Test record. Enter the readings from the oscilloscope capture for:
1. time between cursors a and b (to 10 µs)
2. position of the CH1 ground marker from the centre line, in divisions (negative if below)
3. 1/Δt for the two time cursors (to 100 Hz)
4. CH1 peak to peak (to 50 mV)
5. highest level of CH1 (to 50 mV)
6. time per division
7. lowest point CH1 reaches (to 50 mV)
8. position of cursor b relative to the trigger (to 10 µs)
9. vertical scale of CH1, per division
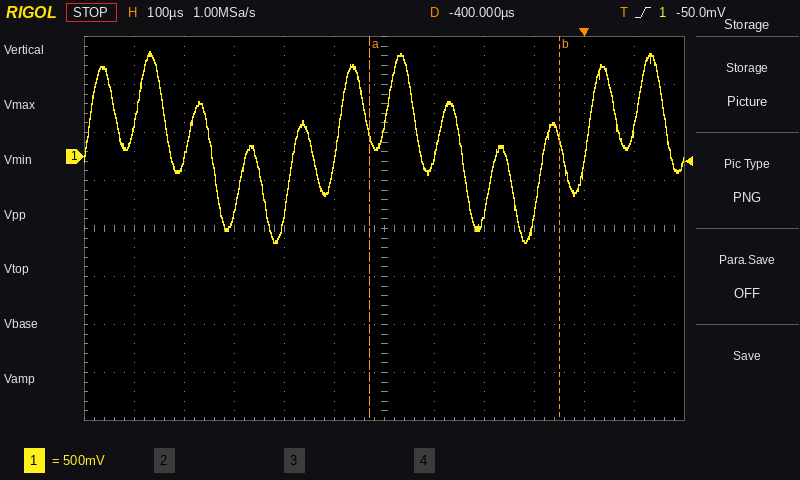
380 µs
+1.5 div
2.6 kHz
2.00 V
1.10 V
100 µs
-900 mV
-50 µs
500 mV
